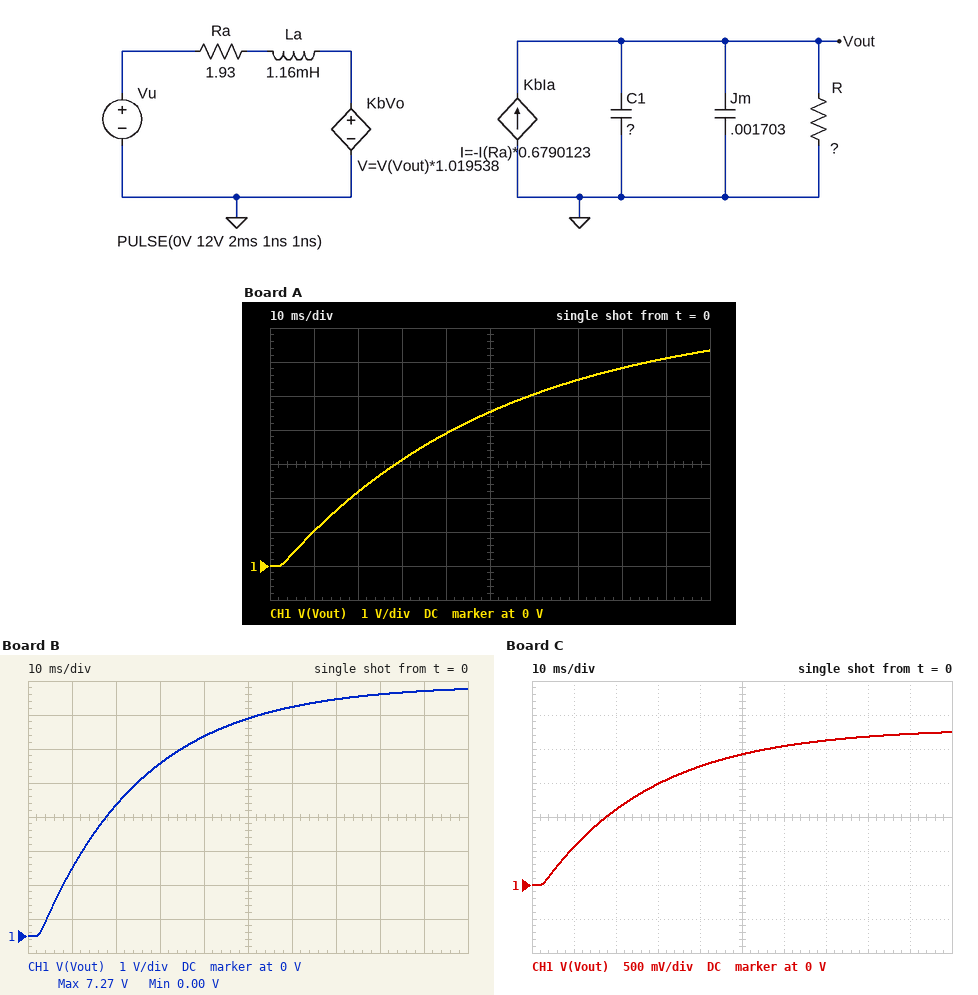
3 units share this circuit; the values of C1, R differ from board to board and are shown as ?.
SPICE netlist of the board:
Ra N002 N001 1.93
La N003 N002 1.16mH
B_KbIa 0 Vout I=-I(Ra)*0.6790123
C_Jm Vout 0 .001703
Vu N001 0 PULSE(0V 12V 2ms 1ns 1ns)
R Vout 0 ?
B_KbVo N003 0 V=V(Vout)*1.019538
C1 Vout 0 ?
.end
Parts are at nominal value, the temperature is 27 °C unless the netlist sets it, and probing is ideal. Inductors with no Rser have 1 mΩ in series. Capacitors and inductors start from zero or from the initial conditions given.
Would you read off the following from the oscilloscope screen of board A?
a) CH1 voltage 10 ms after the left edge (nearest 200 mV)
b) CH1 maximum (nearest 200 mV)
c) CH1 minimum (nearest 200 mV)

1.0 V
6.4 V
0 V
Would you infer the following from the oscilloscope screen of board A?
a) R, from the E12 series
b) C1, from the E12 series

4.7 Ω
27 mF
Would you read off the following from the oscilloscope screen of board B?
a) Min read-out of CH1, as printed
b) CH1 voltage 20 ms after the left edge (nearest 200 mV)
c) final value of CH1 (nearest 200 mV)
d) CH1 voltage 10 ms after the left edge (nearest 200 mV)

0.00 V
3.8 V
7.2 V
2.0 V
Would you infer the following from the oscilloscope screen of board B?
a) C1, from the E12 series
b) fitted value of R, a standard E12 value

12 mF
4.7 Ω
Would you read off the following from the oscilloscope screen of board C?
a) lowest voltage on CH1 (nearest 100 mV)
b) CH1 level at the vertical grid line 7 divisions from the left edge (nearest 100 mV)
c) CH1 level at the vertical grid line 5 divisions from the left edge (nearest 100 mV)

0 V
2.1 V
1.9 V
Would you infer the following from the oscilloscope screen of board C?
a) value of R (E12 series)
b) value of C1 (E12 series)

0.68 Ω
47 mF
